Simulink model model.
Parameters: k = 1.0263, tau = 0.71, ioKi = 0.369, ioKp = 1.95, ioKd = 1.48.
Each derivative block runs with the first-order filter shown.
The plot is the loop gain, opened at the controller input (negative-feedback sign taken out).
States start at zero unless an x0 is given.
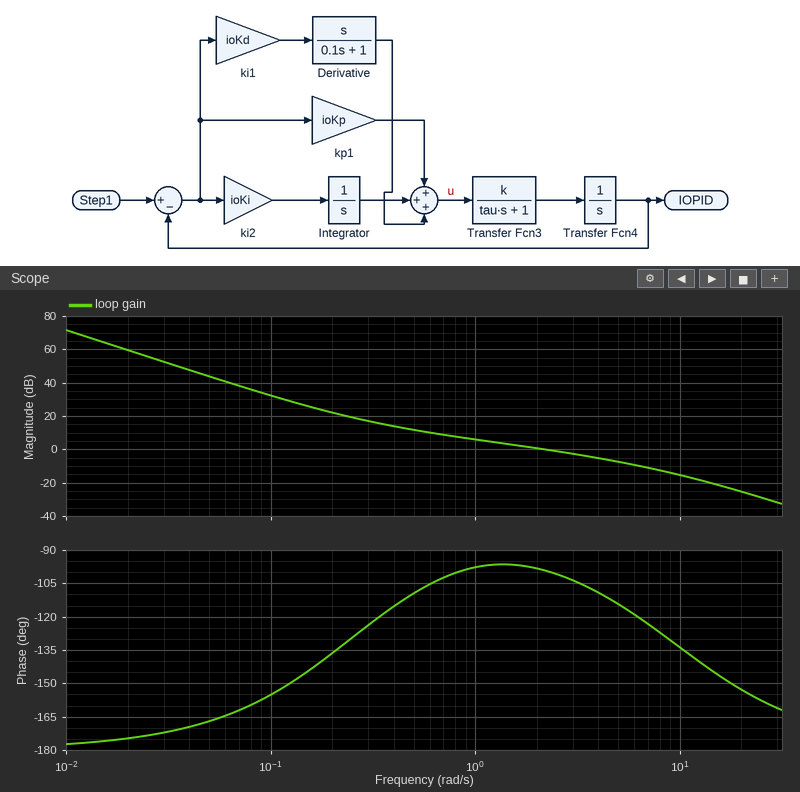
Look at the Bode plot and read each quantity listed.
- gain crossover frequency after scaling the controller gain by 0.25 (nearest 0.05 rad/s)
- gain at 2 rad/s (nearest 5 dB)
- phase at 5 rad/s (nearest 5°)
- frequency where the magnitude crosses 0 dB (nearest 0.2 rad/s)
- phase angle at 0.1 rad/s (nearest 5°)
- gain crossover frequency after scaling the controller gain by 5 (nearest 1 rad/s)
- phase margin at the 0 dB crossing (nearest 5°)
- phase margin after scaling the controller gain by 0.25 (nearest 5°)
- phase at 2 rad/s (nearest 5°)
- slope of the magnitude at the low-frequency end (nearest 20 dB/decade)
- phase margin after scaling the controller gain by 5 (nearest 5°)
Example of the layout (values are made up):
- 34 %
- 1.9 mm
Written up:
- 0.50 rad/s
- 0 dB
- -115°
- 2.2 rad/s
- -155°
- 9 rad/s
- 80°
- 70°
- -100°
- -40 dB/decade
- 50°
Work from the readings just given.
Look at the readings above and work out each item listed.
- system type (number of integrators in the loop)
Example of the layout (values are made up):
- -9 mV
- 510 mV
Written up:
- 2
